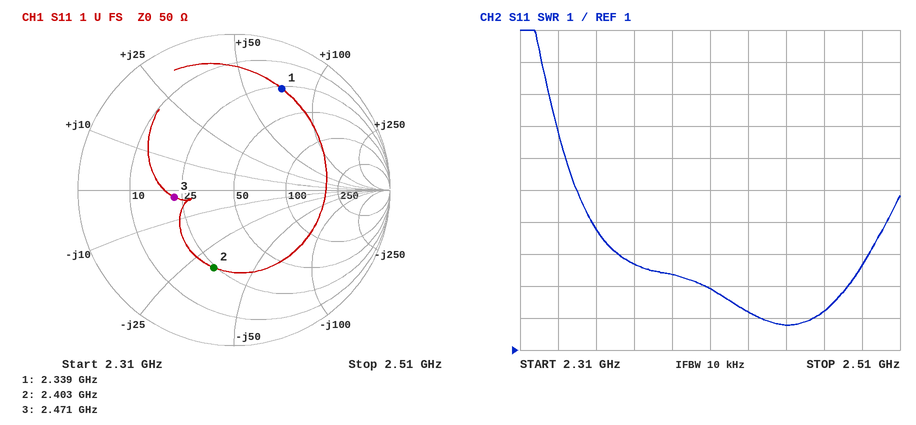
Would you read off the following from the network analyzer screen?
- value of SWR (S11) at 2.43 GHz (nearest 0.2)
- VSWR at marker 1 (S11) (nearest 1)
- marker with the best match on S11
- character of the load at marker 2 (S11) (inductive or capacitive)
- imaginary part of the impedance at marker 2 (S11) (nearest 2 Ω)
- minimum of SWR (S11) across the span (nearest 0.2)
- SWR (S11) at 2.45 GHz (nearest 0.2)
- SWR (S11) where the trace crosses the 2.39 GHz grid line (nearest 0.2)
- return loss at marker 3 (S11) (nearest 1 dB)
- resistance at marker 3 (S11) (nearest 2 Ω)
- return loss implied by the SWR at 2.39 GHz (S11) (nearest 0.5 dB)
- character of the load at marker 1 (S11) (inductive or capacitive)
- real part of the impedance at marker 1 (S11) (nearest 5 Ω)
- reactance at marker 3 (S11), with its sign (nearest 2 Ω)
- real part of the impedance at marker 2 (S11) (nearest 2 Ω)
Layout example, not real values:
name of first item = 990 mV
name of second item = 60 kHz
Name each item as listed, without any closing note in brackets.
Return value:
value of SWR (S11) at 2.43 GHz = 2.2
VSWR at marker 1 (S11) = 6
marker with the best match on S11 = marker 3
character of the load at marker 2 (S11) = capacitive
imaginary part of the impedance at marker 2 (S11) = -32 Ω
minimum of SWR (S11) across the span = 1.8
SWR (S11) at 2.45 GHz = 1.8
SWR (S11) where the trace crosses the 2.39 GHz grid line = 3.4
return loss at marker 3 (S11) = 8 dB
resistance at marker 3 (S11) = 22 Ω
return loss implied by the SWR at 2.39 GHz (S11) = 5.5 dB
character of the load at marker 1 (S11) = inductive
real part of the impedance at marker 1 (S11) = 25 Ω
reactance at marker 3 (S11), with its sign = -2 Ω
real part of the impedance at marker 2 (S11) = 24 Ω
